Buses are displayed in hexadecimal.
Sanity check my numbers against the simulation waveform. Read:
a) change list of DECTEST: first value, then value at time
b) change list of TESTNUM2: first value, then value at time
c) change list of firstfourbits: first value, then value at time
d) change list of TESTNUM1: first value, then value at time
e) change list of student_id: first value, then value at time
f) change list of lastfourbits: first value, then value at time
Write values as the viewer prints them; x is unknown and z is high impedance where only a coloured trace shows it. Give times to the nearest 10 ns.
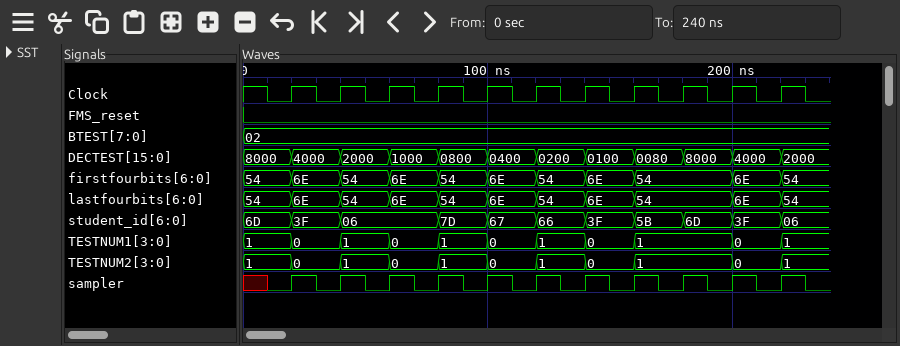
8000, 4000 at 20 ns, 2000 at 40 ns, 1000 at 60 ns, 0800 at 80 ns, 0400 at 100 ns, 0200 at 120 ns, 0100 at 140 ns, 0080 at 160 ns, 8000 at 180 ns, 4000 at 200 ns, 2000 at 220 ns
1, 0 at 20 ns, 1 at 40 ns, 0 at 60 ns, 1 at 80 ns, 0 at 100 ns, 1 at 120 ns, 0 at 140 ns, 1 at 160 ns, 0 at 200 ns, 1 at 220 ns
54, 6E at 20 ns, 54 at 40 ns, 6E at 60 ns, 54 at 80 ns, 6E at 100 ns, 54 at 120 ns, 6E at 140 ns, 54 at 160 ns, 6E at 200 ns, 54 at 220 ns
1, 0 at 20 ns, 1 at 40 ns, 0 at 60 ns, 1 at 80 ns, 0 at 100 ns, 1 at 120 ns, 0 at 140 ns, 1 at 160 ns, 0 at 200 ns, 1 at 220 ns
6D, 3F at 20 ns, 06 at 40 ns, 7D at 80 ns, 67 at 100 ns, 66 at 120 ns, 3F at 140 ns, 5B at 160 ns, 6D at 180 ns, 3F at 200 ns, 06 at 220 ns
54, 6E at 20 ns, 54 at 40 ns, 6E at 60 ns, 54 at 80 ns, 6E at 100 ns, 54 at 120 ns, 6E at 140 ns, 54 at 160 ns, 6E at 200 ns, 54 at 220 ns
